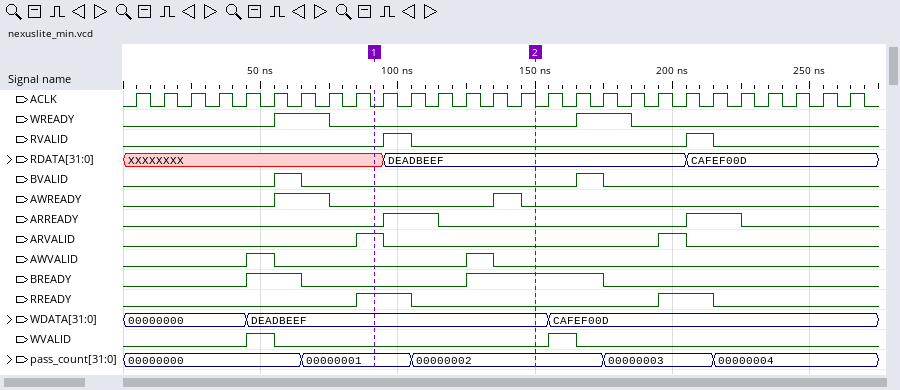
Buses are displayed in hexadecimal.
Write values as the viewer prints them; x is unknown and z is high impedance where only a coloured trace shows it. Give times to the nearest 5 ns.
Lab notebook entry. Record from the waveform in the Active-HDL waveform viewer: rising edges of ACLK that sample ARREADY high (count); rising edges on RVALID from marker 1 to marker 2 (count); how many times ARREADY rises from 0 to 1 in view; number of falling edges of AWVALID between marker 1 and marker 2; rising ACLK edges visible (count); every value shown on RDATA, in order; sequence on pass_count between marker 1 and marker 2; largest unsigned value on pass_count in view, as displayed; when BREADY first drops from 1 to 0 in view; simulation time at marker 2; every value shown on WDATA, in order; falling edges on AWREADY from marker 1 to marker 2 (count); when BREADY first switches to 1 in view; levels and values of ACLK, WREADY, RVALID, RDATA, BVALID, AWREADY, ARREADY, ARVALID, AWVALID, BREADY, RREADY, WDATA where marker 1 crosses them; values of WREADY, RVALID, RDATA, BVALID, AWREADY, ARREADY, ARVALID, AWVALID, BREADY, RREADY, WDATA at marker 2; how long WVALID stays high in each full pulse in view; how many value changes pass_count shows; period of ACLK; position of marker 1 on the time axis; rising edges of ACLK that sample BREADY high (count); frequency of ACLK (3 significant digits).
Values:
4
1
2
1
27
XXXXXXXX, DEADBEEF, CAFEF00D
00000001, 00000002
00000004
65 ns
150 ns
00000000, DEADBEEF, CAFEF00D
1
45 ns
ACLK=0, WREADY=0, RVALID=0, RDATA=XXXXXXXX, BVALID=0, AWREADY=0, ARREADY=0, ARVALID=1, AWVALID=0, BREADY=0, RREADY=1, WDATA=DEADBEEF
WREADY=0, RVALID=0, RDATA=DEADBEEF, BVALID=0, AWREADY=0, ARREADY=0, ARVALID=0, AWVALID=0, BREADY=1, RREADY=0, WDATA=DEADBEEF
10 ns, 10 ns
4
10 ns
90 ns
7
100 MHz
